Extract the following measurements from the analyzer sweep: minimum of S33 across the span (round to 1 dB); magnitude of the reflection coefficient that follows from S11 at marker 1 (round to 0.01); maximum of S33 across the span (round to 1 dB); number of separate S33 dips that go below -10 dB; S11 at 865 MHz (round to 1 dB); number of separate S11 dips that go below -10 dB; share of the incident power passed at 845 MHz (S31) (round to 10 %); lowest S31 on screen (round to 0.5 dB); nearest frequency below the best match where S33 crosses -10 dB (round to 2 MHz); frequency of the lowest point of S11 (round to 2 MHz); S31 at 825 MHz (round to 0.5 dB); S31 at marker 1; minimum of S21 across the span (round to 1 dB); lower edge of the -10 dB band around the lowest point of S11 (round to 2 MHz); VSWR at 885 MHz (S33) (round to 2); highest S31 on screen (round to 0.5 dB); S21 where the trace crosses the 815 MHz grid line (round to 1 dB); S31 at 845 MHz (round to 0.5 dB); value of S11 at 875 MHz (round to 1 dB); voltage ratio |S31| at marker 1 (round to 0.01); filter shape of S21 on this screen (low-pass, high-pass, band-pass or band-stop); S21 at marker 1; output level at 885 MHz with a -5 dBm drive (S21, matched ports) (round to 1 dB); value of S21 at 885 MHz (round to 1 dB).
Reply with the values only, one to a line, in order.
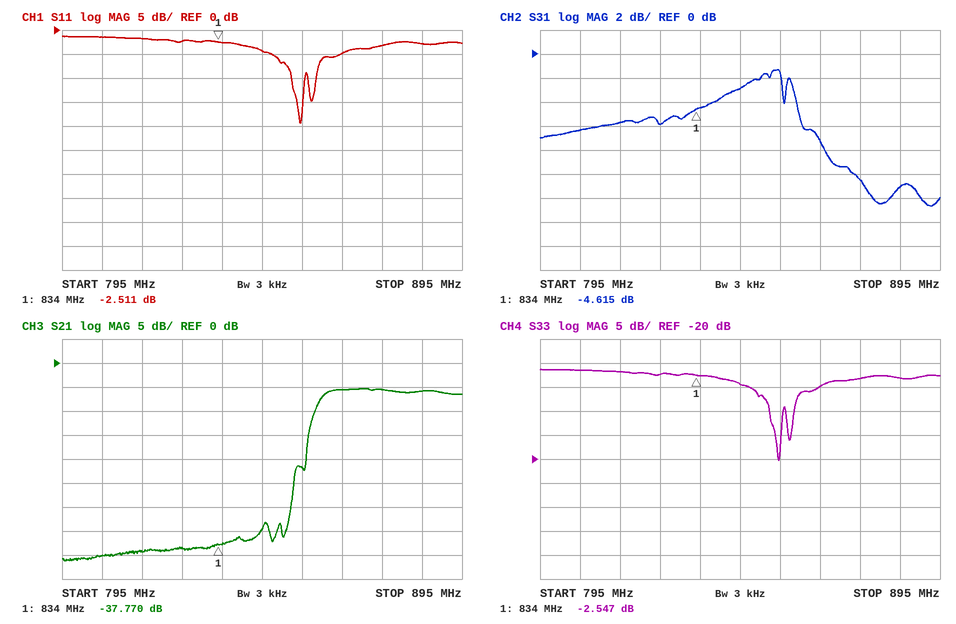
-20 dB
0.75
-1 dB
2
-5 dB
2
50 %
-12.5 dB
852 MHz
854 MHz
-6.0 dB
-4.615 dB
-41 dB
852 MHz
6
-1.5 dB
-39 dB
-3.0 dB
-3 dB
0.59
high-pass
-37.770 dB
-11 dBm
-6 dB
